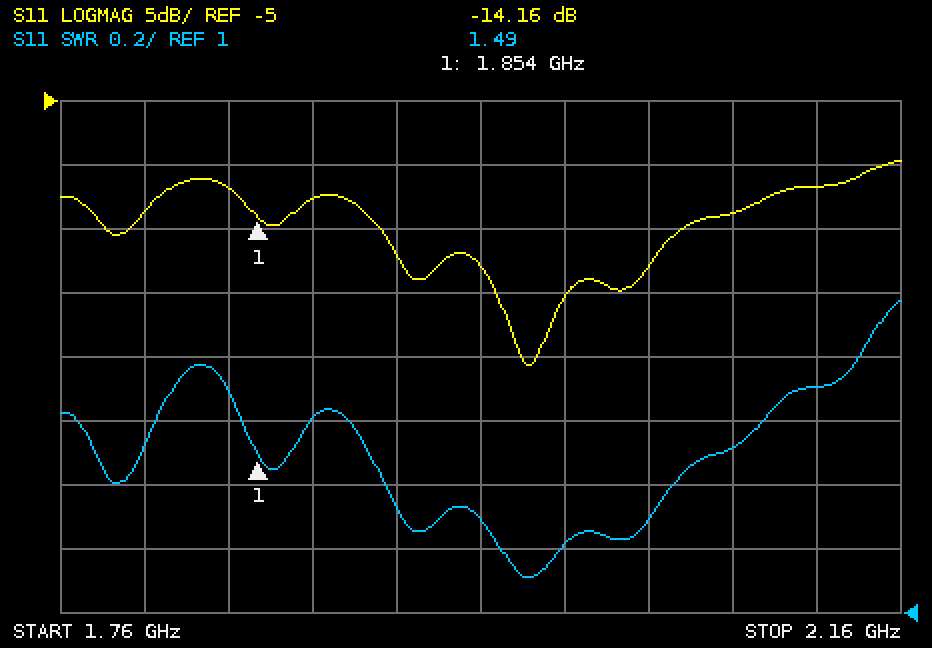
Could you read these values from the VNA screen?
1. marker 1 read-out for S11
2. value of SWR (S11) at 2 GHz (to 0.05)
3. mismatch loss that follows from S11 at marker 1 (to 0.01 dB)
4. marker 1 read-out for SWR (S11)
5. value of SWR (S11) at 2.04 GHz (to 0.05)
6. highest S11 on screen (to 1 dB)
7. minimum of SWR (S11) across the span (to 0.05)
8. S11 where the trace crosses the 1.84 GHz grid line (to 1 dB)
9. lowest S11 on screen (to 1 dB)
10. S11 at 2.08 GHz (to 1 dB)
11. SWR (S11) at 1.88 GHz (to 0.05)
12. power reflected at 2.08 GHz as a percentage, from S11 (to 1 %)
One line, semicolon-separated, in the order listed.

-14.16 dB; 1.20; 0.17 dB; 1.49; 1.30; -10 dB; 1.10; -12 dB; -26 dB; -14 dB; 1.60; 4 %
